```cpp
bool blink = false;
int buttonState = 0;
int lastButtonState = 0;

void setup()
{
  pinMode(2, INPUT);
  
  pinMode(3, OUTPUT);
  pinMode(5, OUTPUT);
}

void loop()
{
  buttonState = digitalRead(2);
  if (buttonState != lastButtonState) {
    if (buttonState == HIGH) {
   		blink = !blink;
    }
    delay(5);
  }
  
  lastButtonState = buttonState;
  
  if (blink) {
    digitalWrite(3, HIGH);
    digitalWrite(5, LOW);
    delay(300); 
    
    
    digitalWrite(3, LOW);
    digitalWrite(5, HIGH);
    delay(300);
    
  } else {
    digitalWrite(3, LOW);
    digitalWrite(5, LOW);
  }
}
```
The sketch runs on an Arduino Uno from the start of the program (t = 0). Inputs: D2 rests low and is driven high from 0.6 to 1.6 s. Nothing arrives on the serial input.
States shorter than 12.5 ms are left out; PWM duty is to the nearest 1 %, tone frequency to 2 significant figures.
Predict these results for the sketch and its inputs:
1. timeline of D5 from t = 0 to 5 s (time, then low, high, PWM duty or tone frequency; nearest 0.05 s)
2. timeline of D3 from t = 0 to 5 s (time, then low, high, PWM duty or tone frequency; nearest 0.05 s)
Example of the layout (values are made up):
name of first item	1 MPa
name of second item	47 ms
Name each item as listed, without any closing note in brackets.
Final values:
timeline of D5 from t = 0 to 5 s	0 s low; 0.9 s high; 1.2 s low; 1.5 s high; 1.8 s low; 2.1 s high; 2.4 s low; 2.7 s high; 3 s low; 3.3 s high; 3.6 s low; 3.9 s high; 4.2 s low; 4.5 s high; 4.8 s low
timeline of D3 from t = 0 to 5 s	0 s low; 0.6 s high; 0.9 s low; 1.2 s high; 1.5 s low; 1.8 s high; 2.1 s low; 2.4 s high; 2.7 s low; 3 s high; 3.3 s low; 3.6 s high; 3.9 s low; 4.2 s high; 4.5 s low; 4.8 s high
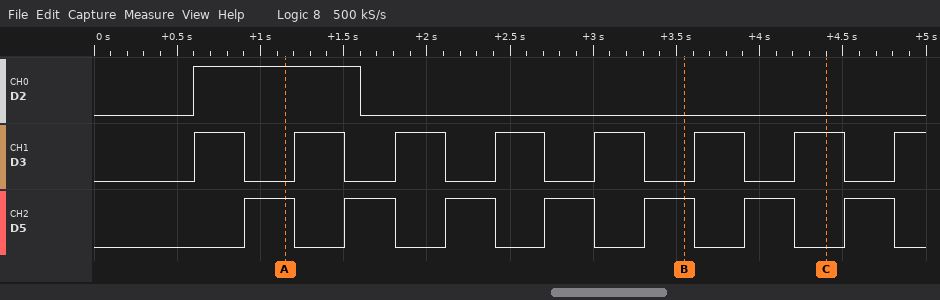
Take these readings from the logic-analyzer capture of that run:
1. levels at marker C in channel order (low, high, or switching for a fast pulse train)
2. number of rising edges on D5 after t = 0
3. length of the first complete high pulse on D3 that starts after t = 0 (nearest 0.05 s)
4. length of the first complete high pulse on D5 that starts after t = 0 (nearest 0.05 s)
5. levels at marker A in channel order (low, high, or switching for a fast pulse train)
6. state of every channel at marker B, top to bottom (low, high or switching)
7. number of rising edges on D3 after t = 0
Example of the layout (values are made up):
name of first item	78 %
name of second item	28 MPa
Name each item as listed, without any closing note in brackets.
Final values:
levels at marker C in channel order	D2 low, D3 high, D5 low
number of rising edges on D5 after t = 0	7
length of the first complete high pulse on D3 that starts after t = 0	0.30 s
length of the first complete high pulse on D5 that starts after t = 0	0.30 s
levels at marker A in channel order	D2 high, D3 low, D5 high
state of every channel at marker B, top to bottom	D2 low, D3 low, D5 high
number of rising edges on D3 after t = 0	8
